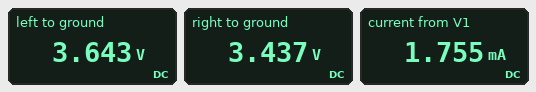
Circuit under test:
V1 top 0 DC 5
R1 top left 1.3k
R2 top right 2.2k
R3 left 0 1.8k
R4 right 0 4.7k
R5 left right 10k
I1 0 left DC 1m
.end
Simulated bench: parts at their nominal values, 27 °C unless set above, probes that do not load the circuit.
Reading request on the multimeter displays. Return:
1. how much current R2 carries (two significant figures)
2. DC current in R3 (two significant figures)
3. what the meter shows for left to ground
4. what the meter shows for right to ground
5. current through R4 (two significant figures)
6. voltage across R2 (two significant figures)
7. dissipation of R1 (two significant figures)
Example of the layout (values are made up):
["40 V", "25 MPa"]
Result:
["710 µA", "2.0 mA", "3.643 V", "3.437 V", "730 µA", "1.6 V", "1.4 mW"]
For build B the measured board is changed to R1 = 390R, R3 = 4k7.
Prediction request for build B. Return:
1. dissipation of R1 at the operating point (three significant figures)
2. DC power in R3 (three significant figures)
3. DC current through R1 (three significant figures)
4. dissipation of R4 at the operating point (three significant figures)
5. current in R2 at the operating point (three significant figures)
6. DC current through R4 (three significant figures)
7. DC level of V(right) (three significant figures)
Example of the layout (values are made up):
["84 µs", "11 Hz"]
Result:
["12.8 µW", "5.17 mW", "181 µA", "2.76 mW", "634 µA", "767 µA", "3.60 V"]
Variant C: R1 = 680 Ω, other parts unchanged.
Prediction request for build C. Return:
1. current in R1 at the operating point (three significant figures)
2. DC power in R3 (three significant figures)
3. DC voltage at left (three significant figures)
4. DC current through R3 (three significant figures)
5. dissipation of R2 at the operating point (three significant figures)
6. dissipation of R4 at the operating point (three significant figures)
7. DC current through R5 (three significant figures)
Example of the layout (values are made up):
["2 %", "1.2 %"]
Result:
["1.33 mA", "9.31 mW", "4.09 V", "2.27 mA", "1.03 mW", "2.60 mW", "59.8 µA"]
